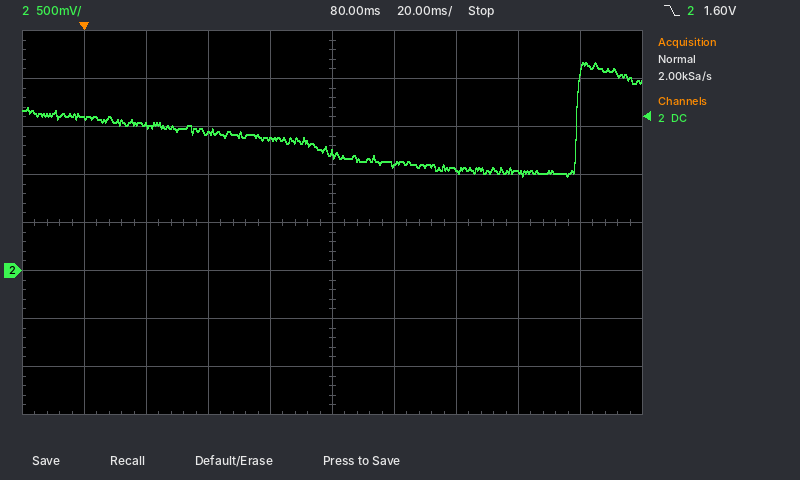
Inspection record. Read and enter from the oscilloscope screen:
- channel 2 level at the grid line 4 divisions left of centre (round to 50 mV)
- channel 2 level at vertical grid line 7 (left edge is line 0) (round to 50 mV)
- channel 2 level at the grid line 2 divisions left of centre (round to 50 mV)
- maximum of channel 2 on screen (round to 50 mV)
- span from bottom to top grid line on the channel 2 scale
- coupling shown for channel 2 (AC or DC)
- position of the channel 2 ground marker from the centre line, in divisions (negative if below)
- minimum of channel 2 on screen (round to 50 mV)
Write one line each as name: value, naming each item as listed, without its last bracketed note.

channel 2 level at the grid line 4 divisions left of centre: 1.60 V
channel 2 level at vertical grid line 7 (left edge is line 0): 1.05 V
channel 2 level at the grid line 2 divisions left of centre: 1.45 V
maximum of channel 2 on screen: 2.15 V
span from bottom to top grid line on the channel 2 scale: 4 V
coupling shown for channel 2: DC
position of the channel 2 ground marker from the centre line, in divisions: -1.0 div
minimum of channel 2 on screen: 1.00 V
